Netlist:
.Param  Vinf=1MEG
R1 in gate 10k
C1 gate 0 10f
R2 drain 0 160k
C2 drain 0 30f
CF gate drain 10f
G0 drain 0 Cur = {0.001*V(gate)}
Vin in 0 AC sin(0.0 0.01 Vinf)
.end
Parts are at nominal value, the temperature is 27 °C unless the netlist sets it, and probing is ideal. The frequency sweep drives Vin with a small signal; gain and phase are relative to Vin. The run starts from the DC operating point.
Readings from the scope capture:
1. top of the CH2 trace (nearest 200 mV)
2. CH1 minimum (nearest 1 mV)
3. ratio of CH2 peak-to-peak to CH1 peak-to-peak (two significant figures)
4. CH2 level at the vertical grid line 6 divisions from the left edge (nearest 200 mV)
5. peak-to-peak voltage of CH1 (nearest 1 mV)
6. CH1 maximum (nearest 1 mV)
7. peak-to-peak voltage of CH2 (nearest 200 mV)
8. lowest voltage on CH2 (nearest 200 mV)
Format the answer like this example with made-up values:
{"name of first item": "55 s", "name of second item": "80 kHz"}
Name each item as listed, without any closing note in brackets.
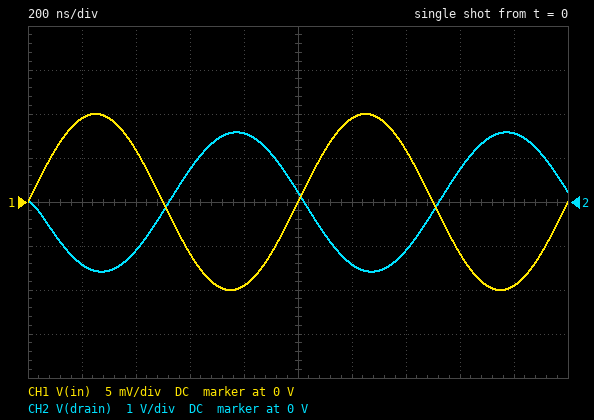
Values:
{"top of the CH2 trace": "1.6 V", "CH1 minimum": "-10 mV", "ratio of CH2 peak-to-peak to CH1 peak-to-peak": "160", "CH2 level at the vertical grid line 6 divisions from the left edge": "-1.4 V", "peak-to-peak voltage of CH1": "20 mV", "CH1 maximum": "10 mV", "peak-to-peak voltage of CH2": "3.2 V", "lowest voltage on CH2": "-1.6 V"}
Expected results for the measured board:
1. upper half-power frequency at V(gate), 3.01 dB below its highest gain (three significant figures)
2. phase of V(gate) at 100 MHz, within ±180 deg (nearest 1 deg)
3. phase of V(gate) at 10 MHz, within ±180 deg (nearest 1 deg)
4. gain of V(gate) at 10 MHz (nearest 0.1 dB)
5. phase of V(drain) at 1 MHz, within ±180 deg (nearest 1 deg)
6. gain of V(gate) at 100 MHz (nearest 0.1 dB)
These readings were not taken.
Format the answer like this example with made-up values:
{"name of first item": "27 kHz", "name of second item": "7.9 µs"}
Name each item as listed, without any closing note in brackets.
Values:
{"upper half-power frequency at V(gate), 3.01 dB below its highest gain": "7.71 MHz", "phase of V(gate) at 100 MHz, within ±180 deg": "-12 deg", "phase of V(gate) at 10 MHz, within ±180 deg": "-33 deg", "gain of V(gate) at 10 MHz": "-4.1 dB", "phase of V(drain) at 1 MHz, within ±180 deg": "172 deg", "gain of V(gate) at 100 MHz": "-10.7 dB"}
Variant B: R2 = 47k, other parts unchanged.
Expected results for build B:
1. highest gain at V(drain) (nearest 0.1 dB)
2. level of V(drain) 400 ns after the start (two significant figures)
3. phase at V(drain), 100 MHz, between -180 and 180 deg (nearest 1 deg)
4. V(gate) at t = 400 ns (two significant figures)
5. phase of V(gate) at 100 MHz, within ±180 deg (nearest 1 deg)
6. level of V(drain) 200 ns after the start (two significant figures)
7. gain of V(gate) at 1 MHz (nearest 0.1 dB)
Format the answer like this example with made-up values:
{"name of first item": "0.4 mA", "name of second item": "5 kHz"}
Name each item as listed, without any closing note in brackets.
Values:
{"highest gain at V(drain)": "33.4 dB", "level of V(drain) 400 ns after the start": "-290 mV", "phase at V(drain), 100 MHz, between -180 and 180 deg": "101 deg", "V(gate) at t = 400 ns": "6.1 mV", "phase of V(gate) at 100 MHz, within ±180 deg": "-29 deg", "level of V(drain) 200 ns after the start": "-440 mV", "gain of V(gate) at 1 MHz": "0 dB"}
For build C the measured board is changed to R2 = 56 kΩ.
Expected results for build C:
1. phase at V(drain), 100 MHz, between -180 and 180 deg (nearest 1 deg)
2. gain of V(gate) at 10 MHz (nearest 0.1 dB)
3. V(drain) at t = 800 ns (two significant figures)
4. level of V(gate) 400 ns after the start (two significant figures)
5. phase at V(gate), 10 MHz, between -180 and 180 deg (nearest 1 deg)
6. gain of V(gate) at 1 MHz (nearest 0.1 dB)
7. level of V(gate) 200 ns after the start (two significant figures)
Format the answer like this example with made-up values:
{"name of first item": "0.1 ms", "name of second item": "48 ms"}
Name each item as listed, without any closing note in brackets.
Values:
{"phase at V(drain), 100 MHz, between -180 and 180 deg": "99 deg", "gain of V(gate) at 10 MHz": "-0.9 dB", "V(drain) at t = 800 ns": "540 mV", "level of V(gate) 400 ns after the start": "6.2 mV", "phase at V(gate), 10 MHz, between -180 and 180 deg": "-19 deg", "gain of V(gate) at 1 MHz": "0 dB", "level of V(gate) 200 ns after the start": "9.4 mV"}
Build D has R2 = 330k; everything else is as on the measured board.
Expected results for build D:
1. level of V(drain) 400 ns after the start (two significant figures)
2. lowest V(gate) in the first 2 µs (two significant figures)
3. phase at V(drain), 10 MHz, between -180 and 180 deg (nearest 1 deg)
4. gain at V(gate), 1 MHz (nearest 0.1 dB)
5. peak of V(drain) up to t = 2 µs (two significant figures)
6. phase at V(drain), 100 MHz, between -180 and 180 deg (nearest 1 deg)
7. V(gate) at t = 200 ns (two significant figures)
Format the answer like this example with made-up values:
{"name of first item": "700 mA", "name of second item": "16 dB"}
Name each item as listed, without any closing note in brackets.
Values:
{"level of V(drain) 400 ns after the start": "-2.5 V", "lowest V(gate) in the first 2 µs": "-9.6 mV", "phase at V(drain), 10 MHz, between -180 and 180 deg": "109 deg", "gain at V(gate), 1 MHz": "-0.3 dB", "peak of V(drain) up to t = 2 µs": "3.2 V", "phase at V(drain), 100 MHz, between -180 and 180 deg": "90 deg", "V(gate) at t = 200 ns": "8.4 mV"}
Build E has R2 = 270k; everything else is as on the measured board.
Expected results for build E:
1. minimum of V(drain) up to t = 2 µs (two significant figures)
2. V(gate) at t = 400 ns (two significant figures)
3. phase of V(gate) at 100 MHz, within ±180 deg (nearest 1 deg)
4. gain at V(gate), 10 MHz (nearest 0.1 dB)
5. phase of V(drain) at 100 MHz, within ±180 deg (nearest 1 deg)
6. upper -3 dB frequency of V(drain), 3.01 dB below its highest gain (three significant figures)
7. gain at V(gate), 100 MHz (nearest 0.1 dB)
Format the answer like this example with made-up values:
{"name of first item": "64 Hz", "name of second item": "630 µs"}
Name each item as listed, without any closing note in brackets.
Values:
{"minimum of V(drain) up to t = 2 µs": "-2.6 V", "V(gate) at t = 400 ns": "7.0 mV", "phase of V(gate) at 100 MHz, within ±180 deg": "-8 deg", "gain at V(gate), 10 MHz": "-6.6 dB", "phase of V(drain) at 100 MHz, within ±180 deg": "90 deg", "upper -3 dB frequency of V(drain), 3.01 dB below its highest gain": "4.19 MHz", "gain at V(gate), 100 MHz": "-10.8 dB"}
